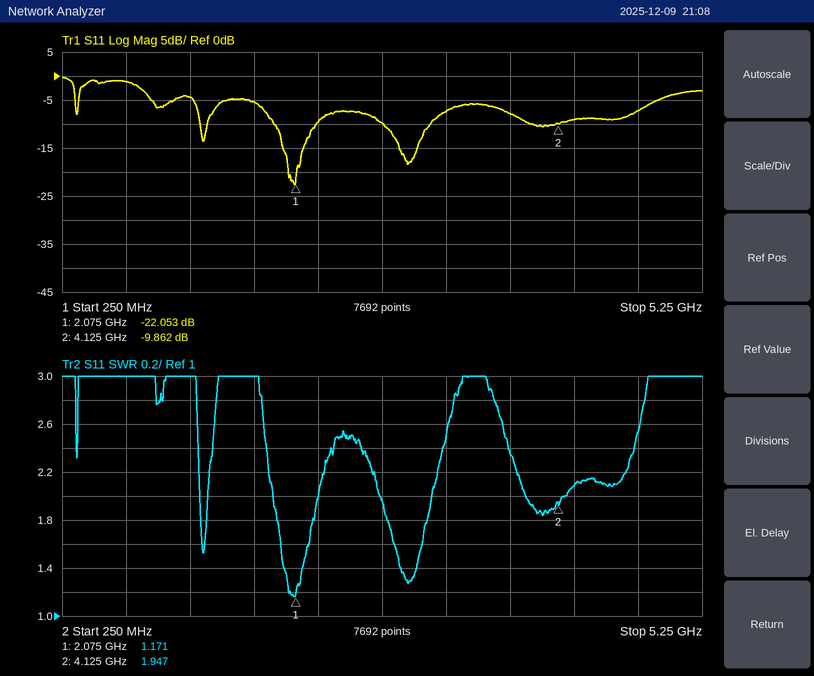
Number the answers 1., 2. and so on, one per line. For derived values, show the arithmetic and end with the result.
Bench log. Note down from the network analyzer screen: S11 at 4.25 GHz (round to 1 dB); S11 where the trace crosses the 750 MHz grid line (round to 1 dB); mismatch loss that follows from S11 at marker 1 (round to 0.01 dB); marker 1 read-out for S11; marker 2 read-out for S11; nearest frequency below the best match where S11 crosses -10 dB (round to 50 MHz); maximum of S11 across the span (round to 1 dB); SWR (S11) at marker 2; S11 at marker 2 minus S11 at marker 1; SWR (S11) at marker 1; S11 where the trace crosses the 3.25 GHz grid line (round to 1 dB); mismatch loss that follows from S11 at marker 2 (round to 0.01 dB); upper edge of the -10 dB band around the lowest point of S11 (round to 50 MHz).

1. -9 dB
2. -1 dB
3. −10 log10(1 − 10^(-22.053/10)) ≈ 0.03 dB
4. -22.053 dB
5. -9.862 dB
6. 1.90 GHz
7. 0 dB
8. 1.947
9. -9.862 − (-22.053) = 12.191 dB
10. 1.171
11. -7 dB
12. −10 log10(1 − 10^(-9.862/10)) ≈ 0.47 dB
13. 2.25 GHz
